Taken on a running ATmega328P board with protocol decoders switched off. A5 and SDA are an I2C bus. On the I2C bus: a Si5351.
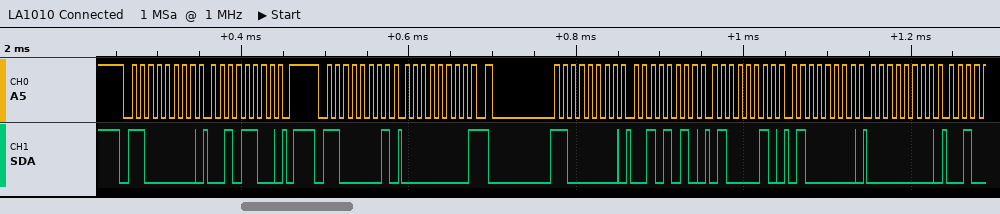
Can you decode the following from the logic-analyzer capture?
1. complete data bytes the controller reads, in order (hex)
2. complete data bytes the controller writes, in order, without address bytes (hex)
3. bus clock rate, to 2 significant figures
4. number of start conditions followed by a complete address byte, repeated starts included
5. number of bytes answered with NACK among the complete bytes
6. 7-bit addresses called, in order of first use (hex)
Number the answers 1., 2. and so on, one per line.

1. 00
2. 2C 2A 42 40 00
3. 100 kHz
4. 3
5. 1
6. 0x60
